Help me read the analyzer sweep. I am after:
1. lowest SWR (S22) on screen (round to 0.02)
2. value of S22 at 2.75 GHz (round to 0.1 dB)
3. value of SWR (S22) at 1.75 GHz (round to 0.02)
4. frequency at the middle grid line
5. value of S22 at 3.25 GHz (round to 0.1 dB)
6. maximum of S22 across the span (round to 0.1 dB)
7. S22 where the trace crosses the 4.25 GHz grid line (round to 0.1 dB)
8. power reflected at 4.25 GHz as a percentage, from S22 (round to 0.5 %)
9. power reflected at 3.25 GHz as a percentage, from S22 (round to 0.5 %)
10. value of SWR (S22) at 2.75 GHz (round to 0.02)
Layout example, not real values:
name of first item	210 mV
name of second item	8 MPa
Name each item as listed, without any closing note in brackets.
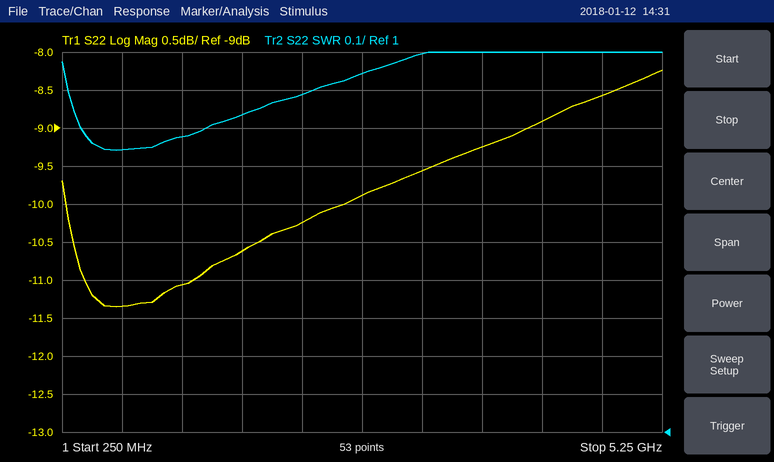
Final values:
lowest SWR (S22) on screen	1.74
value of S22 at 2.75 GHz	-9.9 dB
value of SWR (S22) at 1.75 GHz	1.84
frequency at the middle grid line	2.75 GHz
value of S22 at 3.25 GHz	-9.6 dB
maximum of S22 across the span	-8.2 dB
S22 where the trace crosses the 4.25 GHz grid line	-8.9 dB
power reflected at 4.25 GHz as a percentage, from S22	13.0 %
power reflected at 3.25 GHz as a percentage, from S22	11.0 %
value of SWR (S22) at 2.75 GHz	1.94
